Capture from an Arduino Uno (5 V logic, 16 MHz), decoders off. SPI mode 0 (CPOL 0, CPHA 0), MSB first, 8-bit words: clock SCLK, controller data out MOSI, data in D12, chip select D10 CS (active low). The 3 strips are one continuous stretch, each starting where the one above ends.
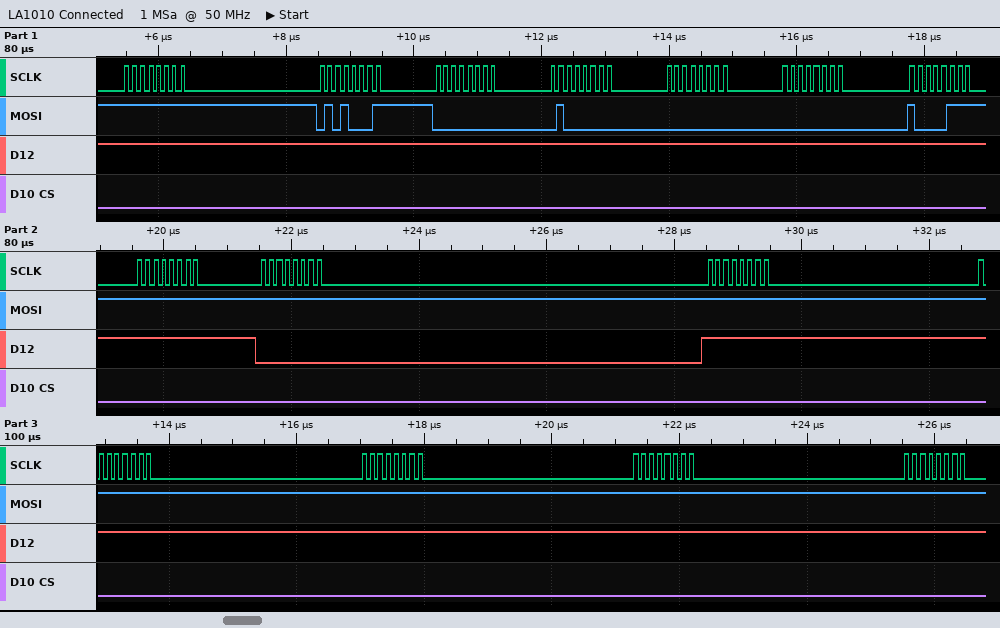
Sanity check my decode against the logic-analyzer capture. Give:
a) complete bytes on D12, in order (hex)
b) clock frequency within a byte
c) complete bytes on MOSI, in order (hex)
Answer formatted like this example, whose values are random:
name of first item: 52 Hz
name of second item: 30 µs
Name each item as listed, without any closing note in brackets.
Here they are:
complete bytes on D12, in order: FF FF FF FF FF FF FF FF 00 FF FF FF FF FF
clock frequency within a byte: 8 MHz
complete bytes on MOSI, in order: FF 51 00 40 00 00 87 FF FF FF FF FF FF FF
